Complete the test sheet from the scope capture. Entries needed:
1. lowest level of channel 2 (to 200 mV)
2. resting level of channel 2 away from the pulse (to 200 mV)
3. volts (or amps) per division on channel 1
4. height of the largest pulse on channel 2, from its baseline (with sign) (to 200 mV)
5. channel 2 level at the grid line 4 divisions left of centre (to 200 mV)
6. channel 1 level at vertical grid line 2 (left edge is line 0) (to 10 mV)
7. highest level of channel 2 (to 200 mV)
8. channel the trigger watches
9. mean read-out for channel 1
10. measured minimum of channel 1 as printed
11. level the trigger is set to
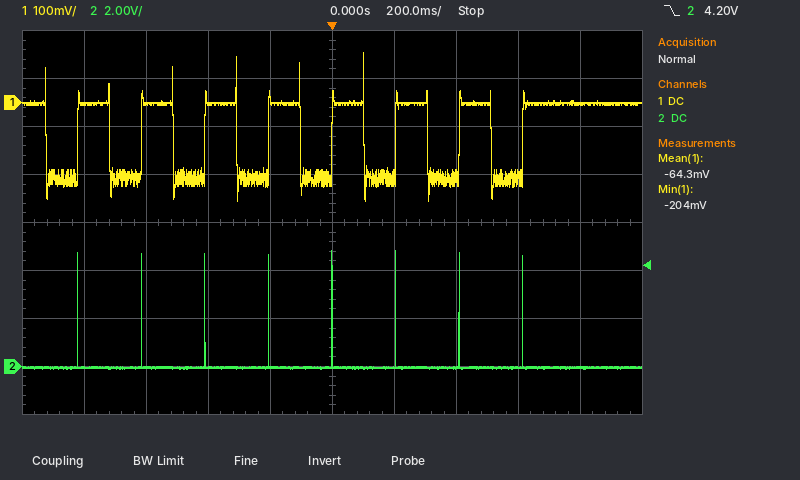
0.0 V
0.0 V
100 mV
+4.8 V
0.0 V
0 mV
4.8 V
channel 2
-64.3 mV
-204 mV
4.20 V
